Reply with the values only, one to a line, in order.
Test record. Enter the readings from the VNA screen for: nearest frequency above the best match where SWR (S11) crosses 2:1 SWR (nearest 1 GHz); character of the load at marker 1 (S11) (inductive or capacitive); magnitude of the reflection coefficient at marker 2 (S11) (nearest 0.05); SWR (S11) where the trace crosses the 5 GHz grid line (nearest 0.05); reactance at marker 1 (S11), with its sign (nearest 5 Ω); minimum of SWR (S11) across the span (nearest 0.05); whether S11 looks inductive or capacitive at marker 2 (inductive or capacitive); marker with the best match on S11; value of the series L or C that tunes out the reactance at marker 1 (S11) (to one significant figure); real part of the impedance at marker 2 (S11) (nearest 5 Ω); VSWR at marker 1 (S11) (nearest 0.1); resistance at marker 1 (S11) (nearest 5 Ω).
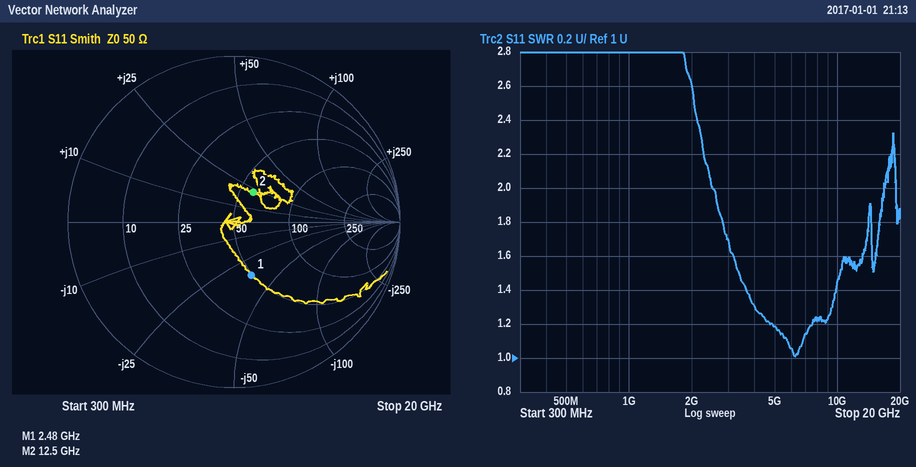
17 GHz
capacitive
0.20
1.20
-35 Ω
1.00
inductive
marker 2
2 nH
60 Ω
2.0
50 Ω
